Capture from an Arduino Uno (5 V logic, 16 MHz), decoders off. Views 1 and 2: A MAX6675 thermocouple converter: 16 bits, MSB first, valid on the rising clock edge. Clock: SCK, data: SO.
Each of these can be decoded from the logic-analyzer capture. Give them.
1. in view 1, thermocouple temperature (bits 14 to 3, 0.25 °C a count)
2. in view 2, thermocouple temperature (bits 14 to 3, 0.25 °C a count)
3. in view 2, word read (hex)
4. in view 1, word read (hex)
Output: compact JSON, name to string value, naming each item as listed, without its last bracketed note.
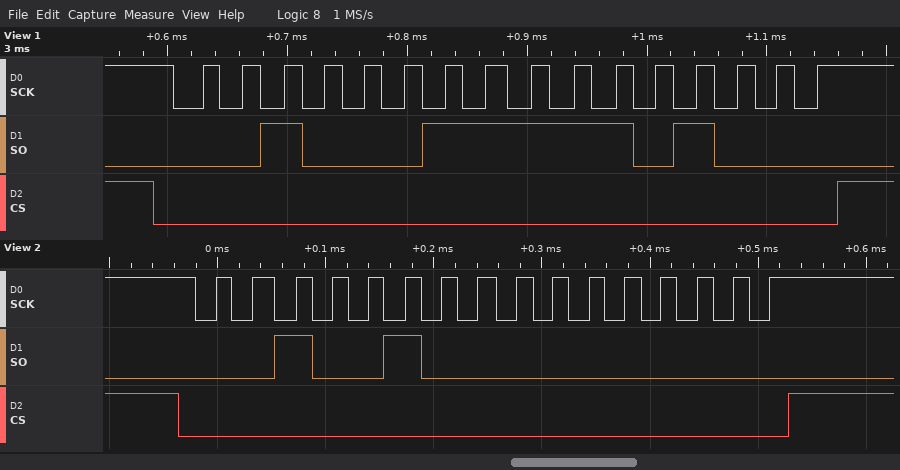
{"in view 1, thermocouple temperature": "287.25 °C", "in view 2, thermocouple temperature": "288.00 °C", "in view 2, word read": "0x2400", "in view 1, word read": "0x23E8"}
